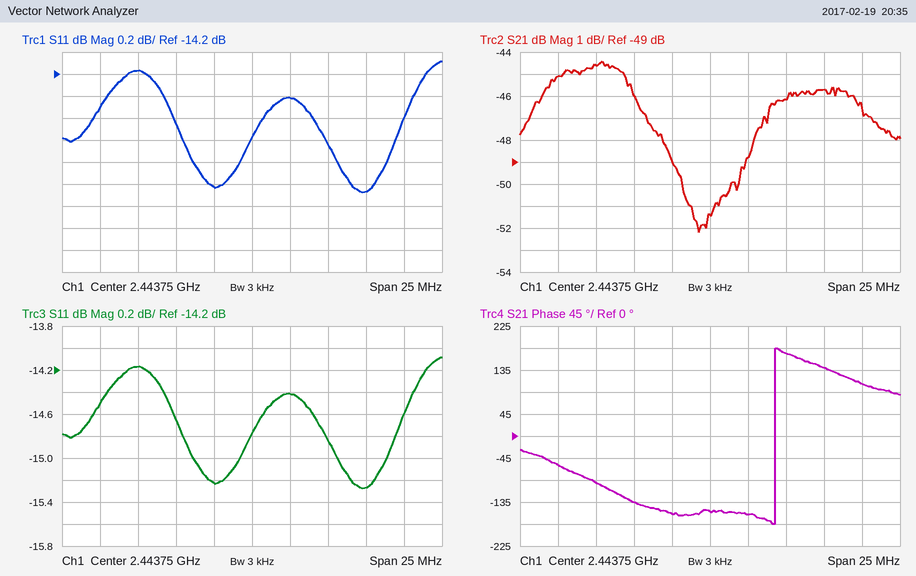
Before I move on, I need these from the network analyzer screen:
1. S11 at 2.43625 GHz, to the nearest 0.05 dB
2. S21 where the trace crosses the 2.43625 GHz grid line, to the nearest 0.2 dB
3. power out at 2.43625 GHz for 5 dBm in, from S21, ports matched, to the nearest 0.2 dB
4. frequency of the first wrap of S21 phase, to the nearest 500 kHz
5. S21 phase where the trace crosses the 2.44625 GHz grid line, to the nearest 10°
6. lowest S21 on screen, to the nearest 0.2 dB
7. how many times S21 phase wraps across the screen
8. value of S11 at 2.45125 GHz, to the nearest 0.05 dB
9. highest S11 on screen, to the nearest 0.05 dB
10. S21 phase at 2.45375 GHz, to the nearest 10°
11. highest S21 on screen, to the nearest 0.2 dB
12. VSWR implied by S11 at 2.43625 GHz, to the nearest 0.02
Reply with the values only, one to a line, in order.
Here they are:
-14.15 dB
-44.6 dB
-39.6 dBm
2.4480 GHz
-160°
-52.2 dB
1
-15.25 dB
-14.10 dB
110°
-44.4 dB
1.48
